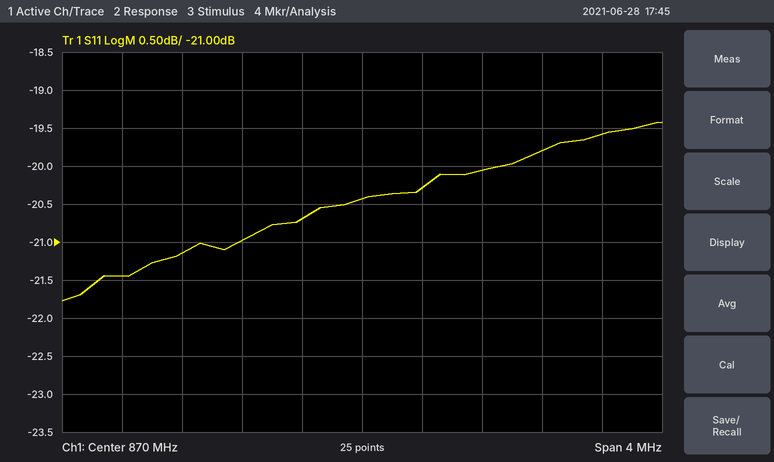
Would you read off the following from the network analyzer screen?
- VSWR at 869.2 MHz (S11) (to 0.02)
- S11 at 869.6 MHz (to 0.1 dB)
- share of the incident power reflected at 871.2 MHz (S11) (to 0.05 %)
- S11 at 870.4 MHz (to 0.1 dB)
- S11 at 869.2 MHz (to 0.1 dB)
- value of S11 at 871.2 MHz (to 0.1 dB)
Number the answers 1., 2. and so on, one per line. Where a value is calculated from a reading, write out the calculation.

1. |Γ| = 10^(-21/20) = 0.0891; VSWR = (1 + 0.0891)/(1 − 0.0891) ≈ 1.20
2. -20.7 dB
3. 10^(-19.8/10) ≈ 1.05 %
4. -20.3 dB
5. -21.0 dB
6. -19.8 dB
